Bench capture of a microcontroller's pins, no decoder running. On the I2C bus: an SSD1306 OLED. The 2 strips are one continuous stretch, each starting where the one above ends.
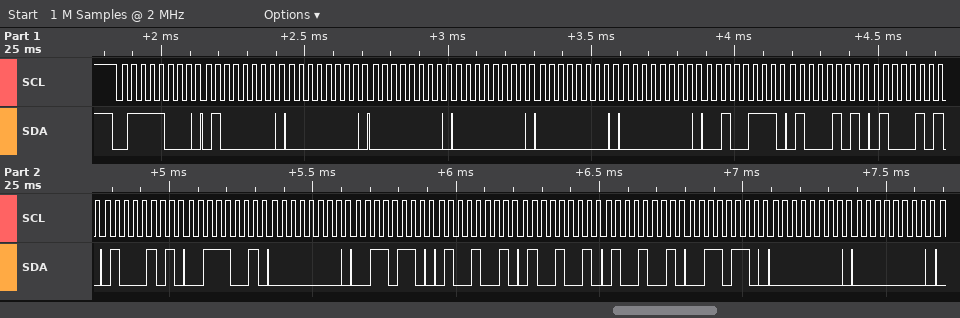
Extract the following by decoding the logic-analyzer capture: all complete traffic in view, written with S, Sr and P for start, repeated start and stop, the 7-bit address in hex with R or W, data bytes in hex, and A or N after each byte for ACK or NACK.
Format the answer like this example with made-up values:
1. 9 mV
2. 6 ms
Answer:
1. S 3CW A 40 A 00 A 00 A 00 A 00 A 00 A 27 A 45 A 45 A 45 A 39 A 00 A 36 A 49 A 49 A 49 A 36 A 00 A 00 A
